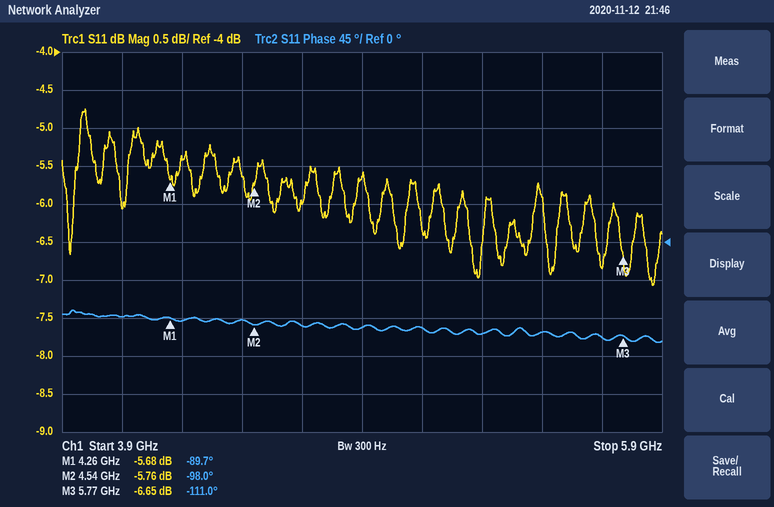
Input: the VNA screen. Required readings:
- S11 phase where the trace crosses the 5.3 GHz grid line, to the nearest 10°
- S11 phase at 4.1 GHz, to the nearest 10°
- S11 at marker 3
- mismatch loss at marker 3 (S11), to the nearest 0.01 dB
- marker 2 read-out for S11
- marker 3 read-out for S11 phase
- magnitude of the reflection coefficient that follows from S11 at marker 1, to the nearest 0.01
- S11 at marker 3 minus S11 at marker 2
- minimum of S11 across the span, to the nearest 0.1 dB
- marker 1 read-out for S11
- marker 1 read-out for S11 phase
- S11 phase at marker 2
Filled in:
-110°
-90°
-6.65 dB
1.06 dB
-5.76 dB
-111.0°
0.52
-0.89 dB
-7.1 dB
-5.68 dB
-89.7°
-98.0°
